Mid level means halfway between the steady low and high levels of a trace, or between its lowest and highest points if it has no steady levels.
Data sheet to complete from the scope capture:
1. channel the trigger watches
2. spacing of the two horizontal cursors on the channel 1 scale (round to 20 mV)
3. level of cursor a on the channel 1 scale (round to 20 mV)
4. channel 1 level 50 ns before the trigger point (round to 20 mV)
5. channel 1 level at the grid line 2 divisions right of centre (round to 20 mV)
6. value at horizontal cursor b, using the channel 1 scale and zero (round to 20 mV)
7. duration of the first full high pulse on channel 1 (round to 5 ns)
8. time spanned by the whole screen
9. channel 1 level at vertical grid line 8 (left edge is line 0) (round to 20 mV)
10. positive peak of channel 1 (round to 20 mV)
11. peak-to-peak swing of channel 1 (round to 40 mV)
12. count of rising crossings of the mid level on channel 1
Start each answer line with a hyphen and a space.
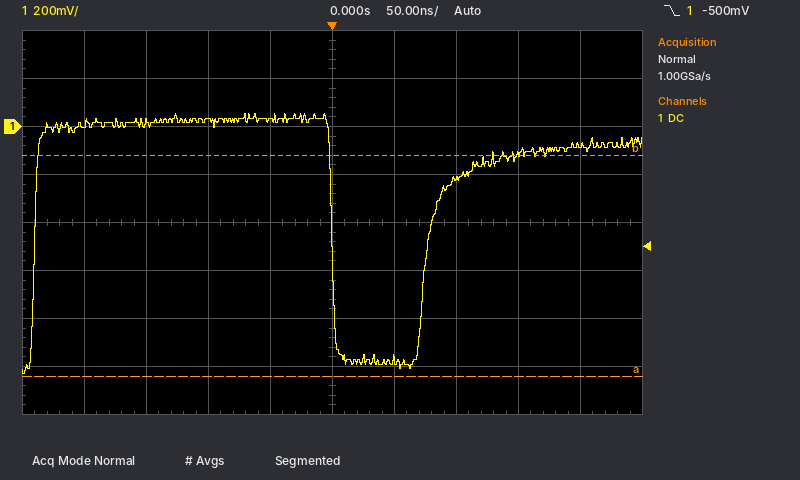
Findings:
- channel 1
- 920 mV
- -1.04 V
- 20 mV
- -220 mV
- -120 mV
- 240 ns
- 500 ns
- -120 mV
- 60 mV
- 1.08 V
- 2
